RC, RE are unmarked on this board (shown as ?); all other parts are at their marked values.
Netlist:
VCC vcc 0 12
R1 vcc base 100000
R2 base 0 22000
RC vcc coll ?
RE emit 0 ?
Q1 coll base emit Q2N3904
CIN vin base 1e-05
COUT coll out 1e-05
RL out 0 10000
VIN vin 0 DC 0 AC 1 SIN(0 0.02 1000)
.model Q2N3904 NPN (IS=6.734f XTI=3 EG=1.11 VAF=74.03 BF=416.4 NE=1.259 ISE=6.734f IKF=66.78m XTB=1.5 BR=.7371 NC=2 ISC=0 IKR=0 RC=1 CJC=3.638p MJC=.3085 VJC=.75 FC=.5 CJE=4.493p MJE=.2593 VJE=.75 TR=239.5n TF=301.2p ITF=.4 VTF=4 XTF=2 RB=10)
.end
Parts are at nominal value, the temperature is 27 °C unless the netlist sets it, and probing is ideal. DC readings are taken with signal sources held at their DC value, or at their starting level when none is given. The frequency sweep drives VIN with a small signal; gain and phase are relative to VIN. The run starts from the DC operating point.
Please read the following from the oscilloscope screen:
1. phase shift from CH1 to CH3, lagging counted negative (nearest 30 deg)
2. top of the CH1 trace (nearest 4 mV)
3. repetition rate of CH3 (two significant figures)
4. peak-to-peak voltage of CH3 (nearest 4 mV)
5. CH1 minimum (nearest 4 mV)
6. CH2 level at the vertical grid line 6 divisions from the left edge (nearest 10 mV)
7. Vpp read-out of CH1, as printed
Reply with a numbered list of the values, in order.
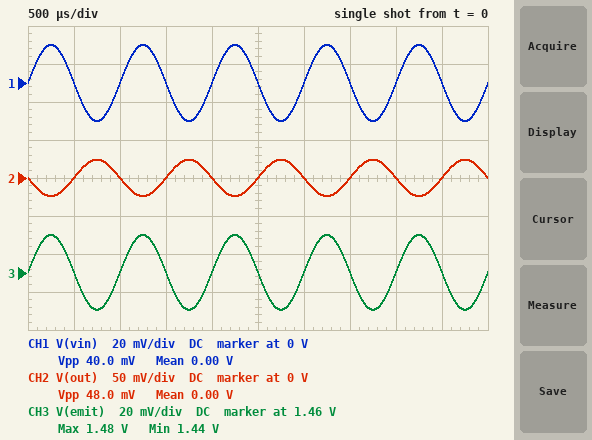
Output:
1. 0 deg
2. 20 mV
3. 1.0 kHz
4. 40 mV
5. -20 mV
6. 0 V
7. 40.0 mV
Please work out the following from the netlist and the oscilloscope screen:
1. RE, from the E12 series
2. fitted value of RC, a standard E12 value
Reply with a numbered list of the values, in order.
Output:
1. 3.3 kΩ
2. 6.8 kΩ
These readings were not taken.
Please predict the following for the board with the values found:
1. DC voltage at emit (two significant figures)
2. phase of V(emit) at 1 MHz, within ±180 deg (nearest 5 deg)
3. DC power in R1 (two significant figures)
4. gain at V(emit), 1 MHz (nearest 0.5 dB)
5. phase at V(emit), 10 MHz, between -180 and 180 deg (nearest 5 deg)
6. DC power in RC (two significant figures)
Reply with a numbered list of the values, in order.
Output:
1. 1.5 V
2. 0 deg
3. 980 µW
4. 0 dB
5. 0 deg
6. 1.3 mW
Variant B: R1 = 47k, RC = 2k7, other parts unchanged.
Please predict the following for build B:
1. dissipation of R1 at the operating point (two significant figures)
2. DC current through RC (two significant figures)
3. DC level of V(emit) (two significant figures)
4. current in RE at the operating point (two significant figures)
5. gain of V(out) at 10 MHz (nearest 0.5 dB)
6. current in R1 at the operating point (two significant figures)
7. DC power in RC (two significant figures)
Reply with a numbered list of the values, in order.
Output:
1. 1.5 mW
2. 920 µA
3. 3.1 V
4. 930 µA
5. -3.5 dB
6. 180 µA
7. 2.3 mW
